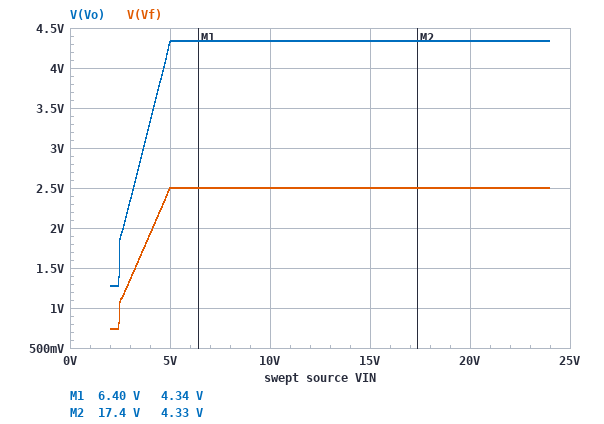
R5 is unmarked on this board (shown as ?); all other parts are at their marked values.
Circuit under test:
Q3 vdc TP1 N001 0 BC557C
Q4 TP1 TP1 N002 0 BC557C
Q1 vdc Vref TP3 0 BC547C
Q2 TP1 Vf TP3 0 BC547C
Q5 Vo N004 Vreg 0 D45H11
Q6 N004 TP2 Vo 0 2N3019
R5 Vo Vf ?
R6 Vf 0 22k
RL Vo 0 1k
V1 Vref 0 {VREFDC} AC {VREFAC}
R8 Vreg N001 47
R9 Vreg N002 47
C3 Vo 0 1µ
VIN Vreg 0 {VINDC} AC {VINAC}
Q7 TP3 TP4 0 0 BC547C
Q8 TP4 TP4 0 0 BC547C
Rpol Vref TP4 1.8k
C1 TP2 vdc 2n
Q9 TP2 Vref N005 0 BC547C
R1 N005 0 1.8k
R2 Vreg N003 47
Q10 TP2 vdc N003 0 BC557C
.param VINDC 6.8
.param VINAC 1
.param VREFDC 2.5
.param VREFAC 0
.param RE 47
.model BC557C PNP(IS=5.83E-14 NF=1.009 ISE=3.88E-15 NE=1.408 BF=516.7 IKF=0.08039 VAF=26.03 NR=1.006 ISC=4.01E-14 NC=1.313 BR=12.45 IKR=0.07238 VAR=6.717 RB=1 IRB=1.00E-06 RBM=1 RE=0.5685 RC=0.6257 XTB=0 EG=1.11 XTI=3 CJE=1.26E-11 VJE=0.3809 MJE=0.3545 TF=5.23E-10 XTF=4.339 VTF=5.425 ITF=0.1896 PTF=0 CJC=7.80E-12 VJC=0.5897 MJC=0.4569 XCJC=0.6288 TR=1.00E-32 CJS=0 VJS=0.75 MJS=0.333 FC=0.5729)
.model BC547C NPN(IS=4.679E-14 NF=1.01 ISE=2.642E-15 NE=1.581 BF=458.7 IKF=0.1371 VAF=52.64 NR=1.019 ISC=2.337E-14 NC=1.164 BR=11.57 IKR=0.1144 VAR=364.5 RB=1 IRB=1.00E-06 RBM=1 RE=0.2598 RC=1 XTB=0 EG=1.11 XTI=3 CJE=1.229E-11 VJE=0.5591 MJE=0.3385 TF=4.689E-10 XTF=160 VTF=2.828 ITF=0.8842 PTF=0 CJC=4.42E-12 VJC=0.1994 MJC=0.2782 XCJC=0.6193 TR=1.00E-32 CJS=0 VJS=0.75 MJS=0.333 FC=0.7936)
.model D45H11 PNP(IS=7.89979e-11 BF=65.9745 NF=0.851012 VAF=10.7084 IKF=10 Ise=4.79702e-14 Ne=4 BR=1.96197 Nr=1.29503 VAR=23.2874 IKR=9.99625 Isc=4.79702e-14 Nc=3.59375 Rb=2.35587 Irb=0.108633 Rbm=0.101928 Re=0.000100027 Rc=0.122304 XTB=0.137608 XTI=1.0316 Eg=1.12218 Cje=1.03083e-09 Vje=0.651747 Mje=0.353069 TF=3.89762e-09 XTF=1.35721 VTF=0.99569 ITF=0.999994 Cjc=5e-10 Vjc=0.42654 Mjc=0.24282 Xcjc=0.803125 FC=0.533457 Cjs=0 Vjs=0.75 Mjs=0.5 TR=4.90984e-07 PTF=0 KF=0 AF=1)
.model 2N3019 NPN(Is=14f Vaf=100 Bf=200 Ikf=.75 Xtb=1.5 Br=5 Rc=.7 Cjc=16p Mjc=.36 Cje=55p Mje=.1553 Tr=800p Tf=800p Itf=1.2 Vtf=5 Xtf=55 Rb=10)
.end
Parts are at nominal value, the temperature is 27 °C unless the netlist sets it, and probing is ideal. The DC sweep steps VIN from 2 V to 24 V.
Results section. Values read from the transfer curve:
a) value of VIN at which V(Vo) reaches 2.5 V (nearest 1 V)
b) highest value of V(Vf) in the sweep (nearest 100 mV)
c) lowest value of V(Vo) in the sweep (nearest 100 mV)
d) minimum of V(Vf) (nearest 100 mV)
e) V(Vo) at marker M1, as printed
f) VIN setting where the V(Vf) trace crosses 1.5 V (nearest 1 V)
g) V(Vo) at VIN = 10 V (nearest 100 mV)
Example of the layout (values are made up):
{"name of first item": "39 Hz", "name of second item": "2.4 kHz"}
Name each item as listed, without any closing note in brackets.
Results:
{"value of VIN at which V(Vo) reaches 2.5 V": "3 V", "highest value of V(Vf) in the sweep": "2.5 V", "lowest value of V(Vo) in the sweep": "1.3 V", "minimum of V(Vf)": "700 mV", "V(Vo) at marker M1, as printed": "4.34 V", "VIN setting where the V(Vf) trace crosses 1.5 V": "3 V", "V(Vo) at VIN = 10 V": "4.3 V"}
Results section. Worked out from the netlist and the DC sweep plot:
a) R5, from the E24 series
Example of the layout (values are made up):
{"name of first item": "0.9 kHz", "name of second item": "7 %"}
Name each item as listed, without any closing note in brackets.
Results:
{"R5, from the E24 series": "16 kΩ"}
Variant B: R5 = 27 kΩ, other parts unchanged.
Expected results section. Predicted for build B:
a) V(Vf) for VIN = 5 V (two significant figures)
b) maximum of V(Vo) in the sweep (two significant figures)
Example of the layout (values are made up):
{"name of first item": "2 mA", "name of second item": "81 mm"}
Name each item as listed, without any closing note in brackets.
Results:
{"V(Vf) for VIN = 5 V": "1.9 V", "maximum of V(Vo) in the sweep": "5.6 V"}
